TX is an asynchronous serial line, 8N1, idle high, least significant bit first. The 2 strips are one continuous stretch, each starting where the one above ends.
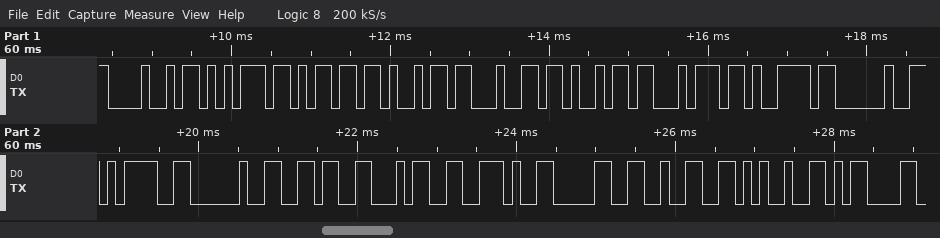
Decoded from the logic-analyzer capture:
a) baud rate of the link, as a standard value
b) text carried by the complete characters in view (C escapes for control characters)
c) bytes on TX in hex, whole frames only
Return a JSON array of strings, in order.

["9600 baud", "\"Humidity = 64.02%\\r\"", "48 75 6D 69 64 69 74 79 20 3D 20 36 34 2E 30 32 25 0D"]
